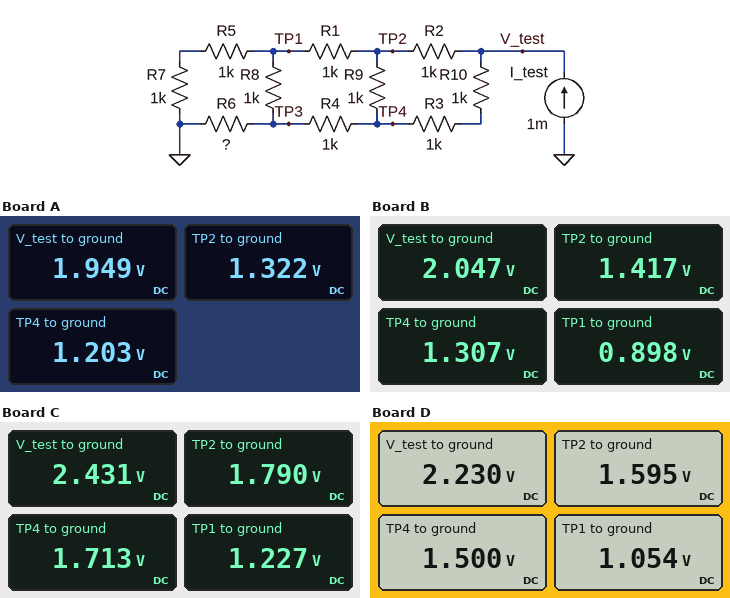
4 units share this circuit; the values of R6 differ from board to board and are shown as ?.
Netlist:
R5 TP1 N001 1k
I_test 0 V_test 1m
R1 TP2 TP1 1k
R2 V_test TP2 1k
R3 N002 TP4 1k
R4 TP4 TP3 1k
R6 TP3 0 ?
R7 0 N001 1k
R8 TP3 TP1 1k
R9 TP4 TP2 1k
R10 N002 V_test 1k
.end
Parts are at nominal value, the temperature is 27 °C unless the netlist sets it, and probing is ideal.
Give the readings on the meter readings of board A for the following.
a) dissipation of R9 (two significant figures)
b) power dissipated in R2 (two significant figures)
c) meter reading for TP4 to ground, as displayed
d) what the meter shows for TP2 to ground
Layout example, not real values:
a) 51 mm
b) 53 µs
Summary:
a) 14 µW
b) 390 µW
c) 1.203 V
d) 1.322 V
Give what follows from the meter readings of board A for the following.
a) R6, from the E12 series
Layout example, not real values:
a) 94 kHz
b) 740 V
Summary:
a) 1.2 kΩ
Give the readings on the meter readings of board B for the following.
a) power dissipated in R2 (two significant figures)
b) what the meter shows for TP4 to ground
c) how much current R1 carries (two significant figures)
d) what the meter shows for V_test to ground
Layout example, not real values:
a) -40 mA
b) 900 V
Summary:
a) 400 µW
b) 1.307 V
c) 520 µA
d) 2.047 V
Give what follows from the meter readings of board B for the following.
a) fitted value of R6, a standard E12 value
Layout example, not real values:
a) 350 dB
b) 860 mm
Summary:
a) 1.5 kΩ
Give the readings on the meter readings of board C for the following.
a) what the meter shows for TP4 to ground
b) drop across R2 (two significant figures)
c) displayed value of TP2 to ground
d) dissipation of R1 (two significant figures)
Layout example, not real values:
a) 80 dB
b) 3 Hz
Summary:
a) 1.713 V
b) 640 mV
c) 1.790 V
d) 320 µW
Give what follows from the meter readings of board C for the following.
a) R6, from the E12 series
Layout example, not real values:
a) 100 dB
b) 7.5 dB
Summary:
a) 3.3 kΩ
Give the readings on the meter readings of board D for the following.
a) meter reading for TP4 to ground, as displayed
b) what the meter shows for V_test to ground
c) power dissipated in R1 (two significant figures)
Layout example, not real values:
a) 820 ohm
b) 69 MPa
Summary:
a) 1.500 V
b) 2.230 V
c) 290 µW
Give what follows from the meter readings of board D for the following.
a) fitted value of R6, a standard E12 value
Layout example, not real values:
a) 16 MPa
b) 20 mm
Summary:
a) 2.2 kΩ
